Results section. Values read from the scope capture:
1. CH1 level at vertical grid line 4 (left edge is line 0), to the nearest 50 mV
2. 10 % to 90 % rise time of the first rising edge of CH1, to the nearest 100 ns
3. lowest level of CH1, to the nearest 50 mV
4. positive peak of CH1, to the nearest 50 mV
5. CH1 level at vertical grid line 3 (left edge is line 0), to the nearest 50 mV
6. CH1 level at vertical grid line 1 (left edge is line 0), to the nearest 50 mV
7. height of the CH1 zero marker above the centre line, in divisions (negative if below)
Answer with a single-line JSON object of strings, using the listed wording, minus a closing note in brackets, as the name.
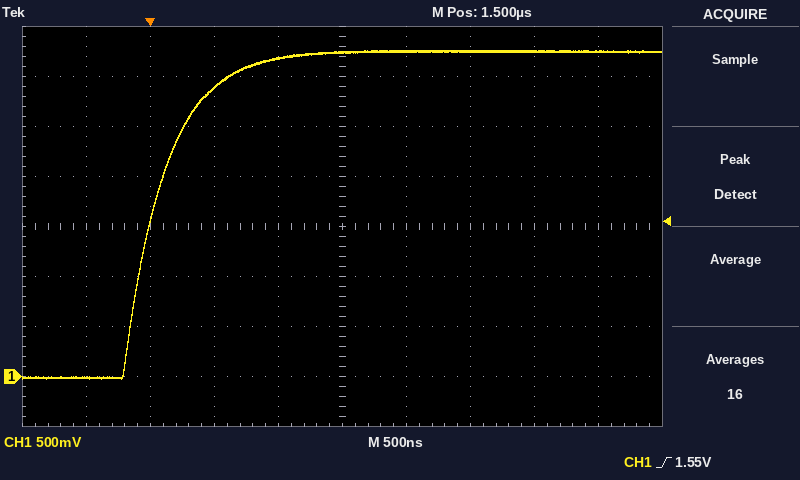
{"CH1 level at vertical grid line 4 (left edge is line 0), to the nearest 50 mV": "3.20 V", "10 % to 90 % rise time of the first rising edge of CH1, to the nearest 100 ns": "700 ns", "lowest level of CH1, to the nearest 50 mV": "0 mV", "positive peak of CH1, to the nearest 50 mV": "3.25 V", "CH1 level at vertical grid line 3 (left edge is line 0), to the nearest 50 mV": "2.90 V", "CH1 level at vertical grid line 1 (left edge is line 0), to the nearest 50 mV": "0 mV", "height of the CH1 zero marker above the centre line, in divisions": "-3.0 div"}
